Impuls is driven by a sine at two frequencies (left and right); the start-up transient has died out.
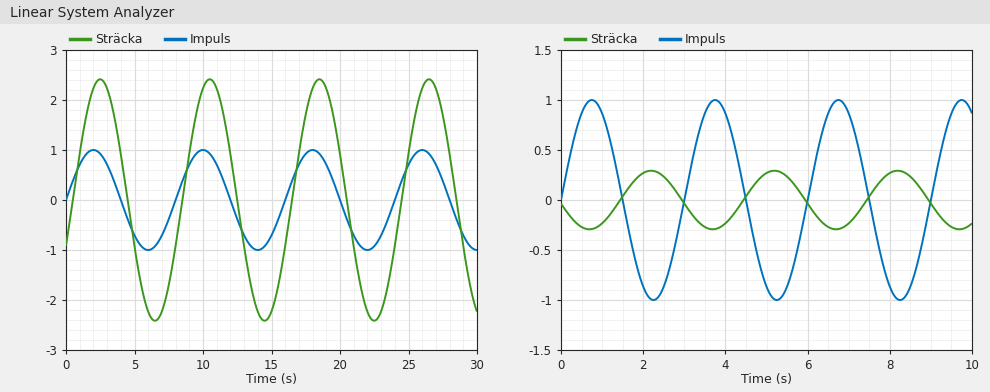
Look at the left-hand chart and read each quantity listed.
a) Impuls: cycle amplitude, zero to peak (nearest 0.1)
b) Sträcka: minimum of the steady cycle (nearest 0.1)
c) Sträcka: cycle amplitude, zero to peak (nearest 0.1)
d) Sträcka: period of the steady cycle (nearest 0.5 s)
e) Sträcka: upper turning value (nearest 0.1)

1.0
-2.4
2.4
8.0 s
2.4
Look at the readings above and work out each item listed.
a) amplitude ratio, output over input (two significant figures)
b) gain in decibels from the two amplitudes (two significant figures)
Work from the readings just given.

2.4
7.6 dB
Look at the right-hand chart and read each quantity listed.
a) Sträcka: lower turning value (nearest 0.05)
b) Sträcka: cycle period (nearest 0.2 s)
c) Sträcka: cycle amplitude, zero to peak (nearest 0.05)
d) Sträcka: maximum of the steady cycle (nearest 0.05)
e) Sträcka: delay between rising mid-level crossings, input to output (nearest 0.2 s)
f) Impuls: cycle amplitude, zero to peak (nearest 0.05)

-0.30
3.0 s
0.30
0.30
1.4 s
1.00
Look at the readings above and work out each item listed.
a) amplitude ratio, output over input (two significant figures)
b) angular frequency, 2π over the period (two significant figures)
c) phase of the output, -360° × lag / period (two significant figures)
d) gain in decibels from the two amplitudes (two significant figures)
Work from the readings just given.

0.30
2.1 rad/s
-170°
-10 dB
